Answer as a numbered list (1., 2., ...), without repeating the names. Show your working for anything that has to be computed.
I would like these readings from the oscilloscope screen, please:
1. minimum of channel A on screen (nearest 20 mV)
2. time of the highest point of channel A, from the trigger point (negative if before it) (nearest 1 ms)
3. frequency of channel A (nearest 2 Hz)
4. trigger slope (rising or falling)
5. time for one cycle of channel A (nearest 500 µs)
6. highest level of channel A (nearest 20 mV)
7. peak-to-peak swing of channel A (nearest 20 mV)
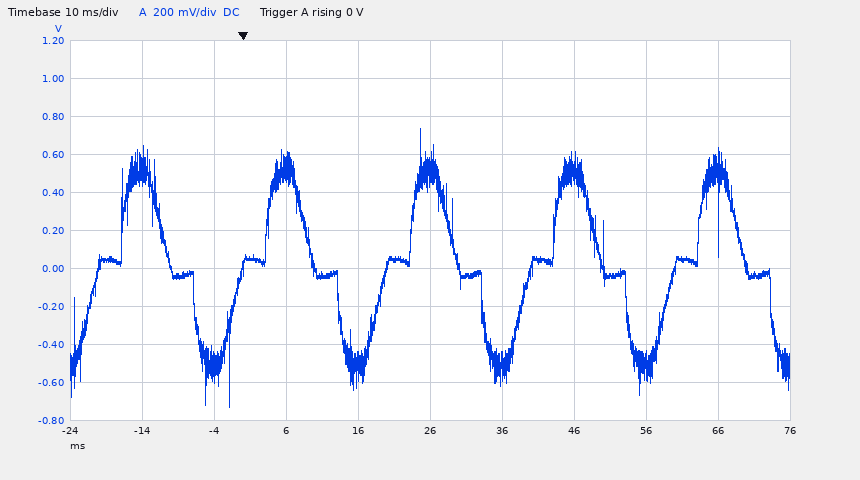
1. -720 mV
2. +25 ms
3. 1 / 20.0 ms ≈ 50 Hz
4. rising
5. 20.0 ms
6. 740 mV
7. 740 mV − (-720 mV) = 1.46 V
